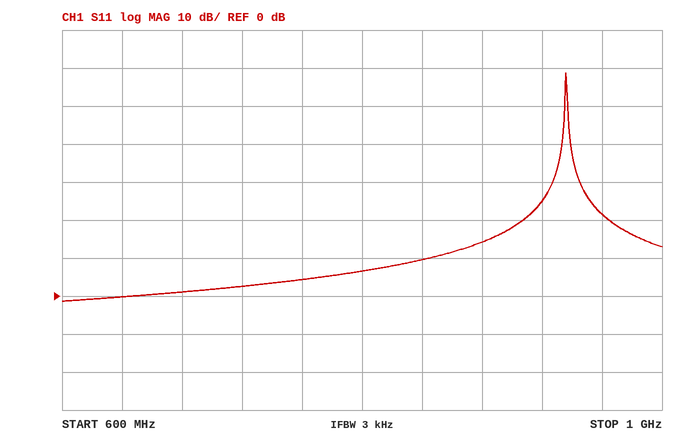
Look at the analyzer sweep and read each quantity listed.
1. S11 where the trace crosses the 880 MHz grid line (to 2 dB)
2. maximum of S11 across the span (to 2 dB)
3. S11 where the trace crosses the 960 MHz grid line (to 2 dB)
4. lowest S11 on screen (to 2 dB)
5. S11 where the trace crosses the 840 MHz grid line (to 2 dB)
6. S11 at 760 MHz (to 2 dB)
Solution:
14 dB
58 dB
22 dB
-2 dB
10 dB
4 dB
